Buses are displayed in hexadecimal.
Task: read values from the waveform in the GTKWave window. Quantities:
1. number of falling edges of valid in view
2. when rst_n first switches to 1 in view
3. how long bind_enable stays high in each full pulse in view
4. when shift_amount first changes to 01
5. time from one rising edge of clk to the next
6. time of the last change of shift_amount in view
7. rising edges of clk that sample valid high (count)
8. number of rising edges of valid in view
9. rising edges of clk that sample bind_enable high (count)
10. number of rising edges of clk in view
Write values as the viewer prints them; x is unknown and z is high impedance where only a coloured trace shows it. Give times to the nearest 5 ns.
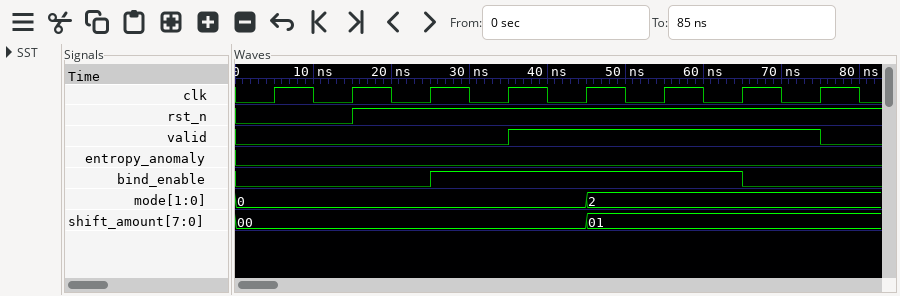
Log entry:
1
15 ns
40 ns
45 ns
10 ns
45 ns
4
1
4
8
